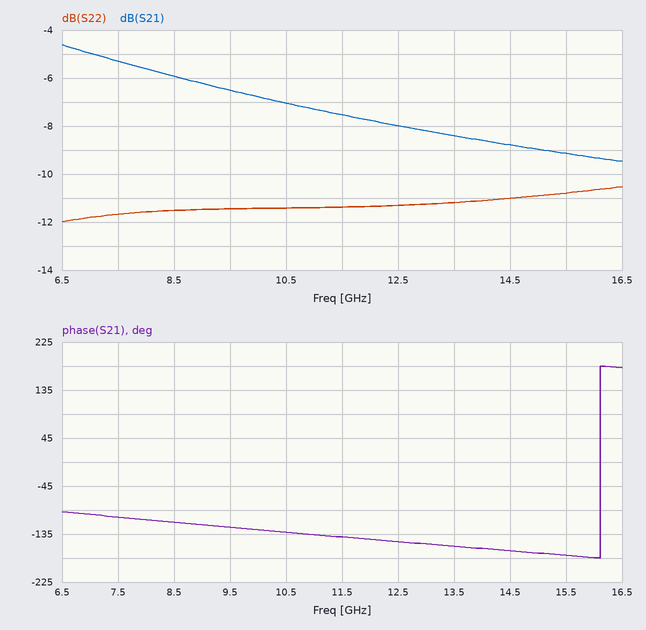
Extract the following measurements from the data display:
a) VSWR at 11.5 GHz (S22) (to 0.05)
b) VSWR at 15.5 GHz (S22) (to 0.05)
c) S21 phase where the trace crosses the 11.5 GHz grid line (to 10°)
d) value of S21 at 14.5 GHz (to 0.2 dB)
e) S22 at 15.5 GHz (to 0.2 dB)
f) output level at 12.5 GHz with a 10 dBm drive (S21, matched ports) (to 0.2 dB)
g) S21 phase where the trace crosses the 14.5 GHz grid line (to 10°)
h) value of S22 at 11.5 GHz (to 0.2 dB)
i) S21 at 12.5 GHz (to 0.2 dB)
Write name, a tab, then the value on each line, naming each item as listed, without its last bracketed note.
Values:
VSWR at 11.5 GHz (S22)	1.75
VSWR at 15.5 GHz (S22)	1.80
S21 phase where the trace crosses the 11.5 GHz grid line	-140°
value of S21 at 14.5 GHz	-8.8 dB
S22 at 15.5 GHz	-10.8 dB
output level at 12.5 GHz with a 10 dBm drive (S21, matched ports)	2.0 dBm
S21 phase where the trace crosses the 14.5 GHz grid line	-170°
value of S22 at 11.5 GHz	-11.4 dB
S21 at 12.5 GHz	-8.0 dB
